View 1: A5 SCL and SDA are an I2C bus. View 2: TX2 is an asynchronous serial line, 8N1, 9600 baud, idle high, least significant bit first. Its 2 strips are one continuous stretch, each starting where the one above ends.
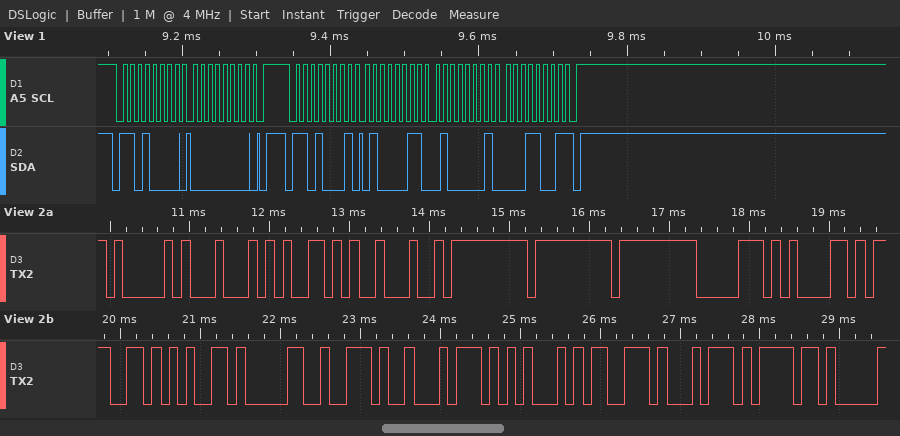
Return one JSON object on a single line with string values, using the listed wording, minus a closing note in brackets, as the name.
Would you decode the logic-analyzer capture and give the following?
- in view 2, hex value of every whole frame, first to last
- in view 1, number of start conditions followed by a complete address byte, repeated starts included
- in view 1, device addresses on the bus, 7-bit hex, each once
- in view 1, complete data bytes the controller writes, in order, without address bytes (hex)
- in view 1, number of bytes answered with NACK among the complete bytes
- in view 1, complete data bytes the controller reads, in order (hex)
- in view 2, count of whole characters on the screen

{"in view 2, hex value of every whole frame, first to last": "41 44 59 22 FF FF FF 70 61 67 65 30 2E 74 45 73 74 6F", "in view 1, number of start conditions followed by a complete address byte, repeated starts included": "2", "in view 1, device addresses on the bus, 7-bit hex, each once": "0x68", "in view 1, complete data bytes the controller writes, in order, without address bytes": "00", "in view 1, number of bytes answered with NACK among the complete bytes": "1", "in view 1, complete data bytes the controller reads, in order": "43 41 19", "in view 2, count of whole characters on the screen": "18"}
